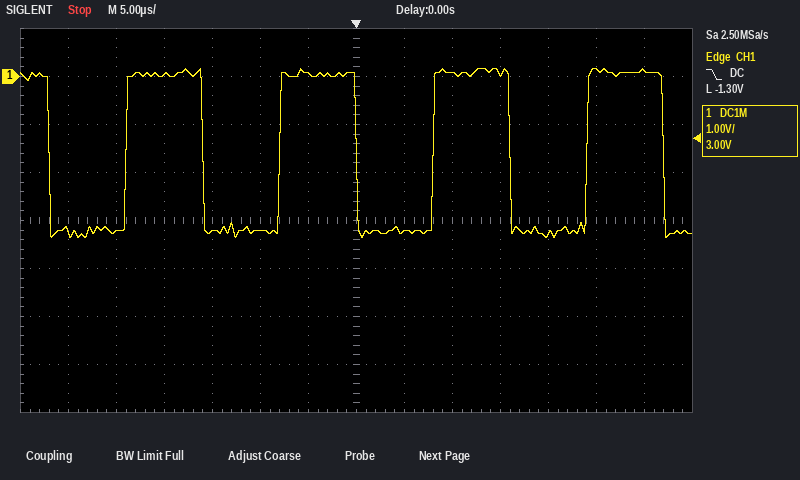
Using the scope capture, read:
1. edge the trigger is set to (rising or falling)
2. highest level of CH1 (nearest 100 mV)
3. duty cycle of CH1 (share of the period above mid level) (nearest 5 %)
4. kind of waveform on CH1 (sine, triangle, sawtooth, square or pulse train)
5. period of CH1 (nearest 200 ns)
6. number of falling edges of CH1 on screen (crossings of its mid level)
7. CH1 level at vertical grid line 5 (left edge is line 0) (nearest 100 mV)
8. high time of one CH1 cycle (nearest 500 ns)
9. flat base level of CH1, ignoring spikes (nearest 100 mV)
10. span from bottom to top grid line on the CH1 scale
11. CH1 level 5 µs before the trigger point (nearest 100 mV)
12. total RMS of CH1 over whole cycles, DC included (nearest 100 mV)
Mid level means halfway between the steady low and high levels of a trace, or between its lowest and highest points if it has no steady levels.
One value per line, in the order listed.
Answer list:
falling
200 mV
50 %
square
16.0 µs
5
-3.2 V
8.0 µs
-3.2 V
8 V
100 mV
2.3 V
